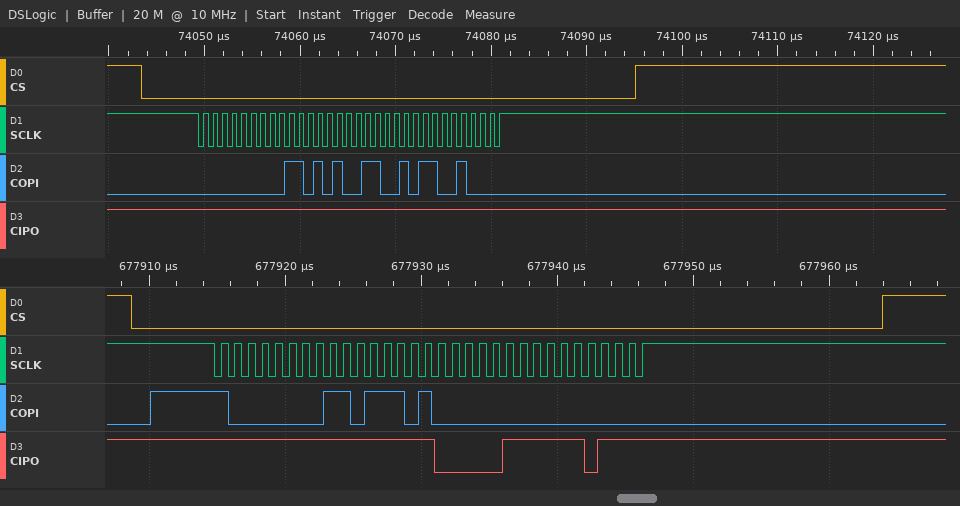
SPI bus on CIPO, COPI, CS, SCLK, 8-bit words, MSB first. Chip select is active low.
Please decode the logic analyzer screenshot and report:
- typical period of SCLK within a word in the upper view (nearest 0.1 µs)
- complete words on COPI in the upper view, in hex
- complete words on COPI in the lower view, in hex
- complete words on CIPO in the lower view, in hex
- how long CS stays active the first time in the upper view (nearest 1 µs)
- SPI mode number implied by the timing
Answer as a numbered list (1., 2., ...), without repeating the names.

1. 1 µs
2. 00, 6A, 65, 90
3. 80, DD, 00, 00
4. FF, FF, 07, EF
5. 52 µs
6. 3
